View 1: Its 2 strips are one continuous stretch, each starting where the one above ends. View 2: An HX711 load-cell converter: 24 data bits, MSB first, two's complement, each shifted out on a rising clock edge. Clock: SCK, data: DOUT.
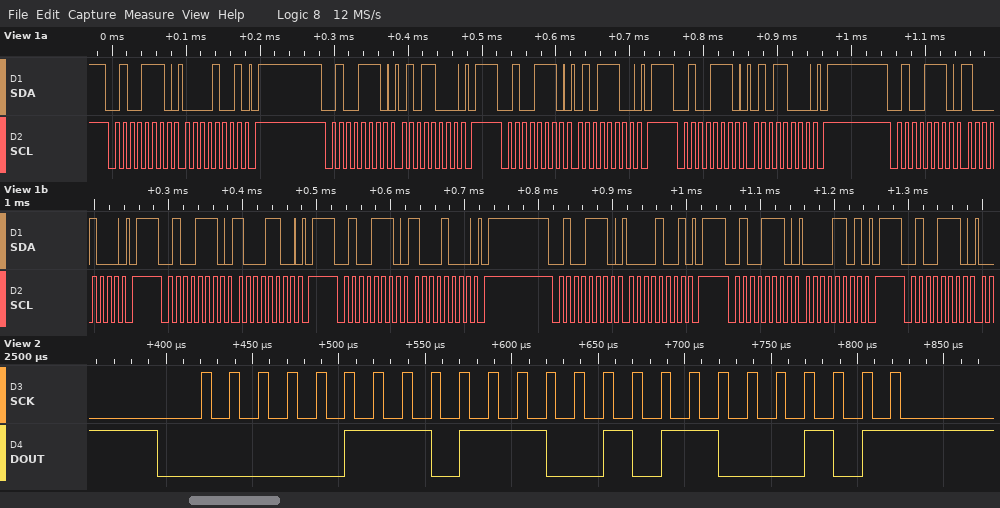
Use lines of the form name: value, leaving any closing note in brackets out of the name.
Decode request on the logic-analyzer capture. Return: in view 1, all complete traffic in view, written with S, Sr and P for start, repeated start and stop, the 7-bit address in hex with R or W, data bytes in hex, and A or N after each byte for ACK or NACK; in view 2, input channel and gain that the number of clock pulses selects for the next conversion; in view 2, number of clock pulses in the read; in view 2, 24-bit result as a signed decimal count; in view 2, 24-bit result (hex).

in view 1, all complete traffic in view, written with S, Sr and P for start, repeated start and stop, the 7-bit address in hex with R or W, data bytes in hex, and A or N after each byte for ACK or NACK: S 27W A 09 A P S 27W A 58 A P S 27W A 5C A P S 27W A 58 A P S 27W A 88 A P S 27W A 8C A P S 27W A 88 A P S 27W A 09 A P S 27W A 0D A P S 27W A
in view 2, input channel and gain that the number of clock pulses selects for the next conversion: channel A, gain 128
in view 2, number of clock pulses in the read: 25
in view 2, 24-bit result as a signed decimal count: 488133
in view 2, 24-bit result: 0x0772C5
